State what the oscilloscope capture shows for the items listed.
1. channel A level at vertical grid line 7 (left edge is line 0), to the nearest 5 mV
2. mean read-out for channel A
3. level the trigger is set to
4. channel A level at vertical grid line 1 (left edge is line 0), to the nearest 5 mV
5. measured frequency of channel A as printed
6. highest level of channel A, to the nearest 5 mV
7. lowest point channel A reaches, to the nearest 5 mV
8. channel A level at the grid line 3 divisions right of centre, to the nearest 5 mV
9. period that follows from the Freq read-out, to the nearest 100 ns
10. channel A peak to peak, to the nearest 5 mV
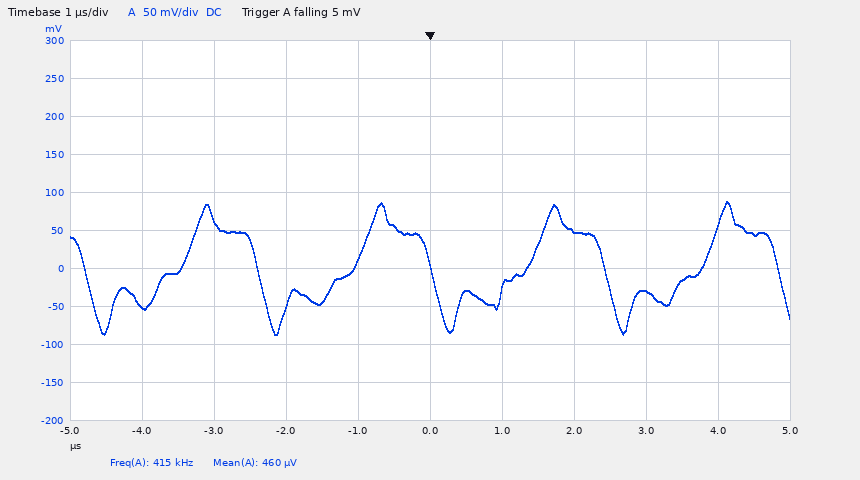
50 mV
460 µV
5 mV
-50 mV
415 kHz
90 mV
-85 mV
-30 mV
2.4 µs
175 mV
